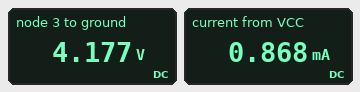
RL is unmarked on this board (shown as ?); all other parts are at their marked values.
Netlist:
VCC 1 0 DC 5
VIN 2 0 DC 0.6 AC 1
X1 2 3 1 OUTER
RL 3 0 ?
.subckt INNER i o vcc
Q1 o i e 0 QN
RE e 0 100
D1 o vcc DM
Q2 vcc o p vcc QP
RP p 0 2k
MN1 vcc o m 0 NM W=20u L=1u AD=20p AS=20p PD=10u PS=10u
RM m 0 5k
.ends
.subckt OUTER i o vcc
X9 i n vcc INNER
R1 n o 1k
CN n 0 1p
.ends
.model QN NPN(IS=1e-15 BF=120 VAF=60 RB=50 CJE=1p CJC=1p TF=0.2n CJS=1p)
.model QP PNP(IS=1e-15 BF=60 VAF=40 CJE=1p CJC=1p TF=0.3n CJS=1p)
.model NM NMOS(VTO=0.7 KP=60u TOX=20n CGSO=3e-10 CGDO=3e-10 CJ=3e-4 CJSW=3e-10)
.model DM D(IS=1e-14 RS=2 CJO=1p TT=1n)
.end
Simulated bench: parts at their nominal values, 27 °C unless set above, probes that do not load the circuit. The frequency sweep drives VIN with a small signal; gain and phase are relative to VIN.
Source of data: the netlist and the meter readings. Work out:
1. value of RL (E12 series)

27 kΩ
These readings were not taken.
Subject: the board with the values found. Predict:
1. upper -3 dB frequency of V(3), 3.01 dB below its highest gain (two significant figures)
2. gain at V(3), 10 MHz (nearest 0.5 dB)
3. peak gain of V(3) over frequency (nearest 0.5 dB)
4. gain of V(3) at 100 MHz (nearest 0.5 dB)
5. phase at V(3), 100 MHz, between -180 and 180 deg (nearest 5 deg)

6.2 GHz
-23.5 dB
-23.0 dB
-26.0 dB
95 deg
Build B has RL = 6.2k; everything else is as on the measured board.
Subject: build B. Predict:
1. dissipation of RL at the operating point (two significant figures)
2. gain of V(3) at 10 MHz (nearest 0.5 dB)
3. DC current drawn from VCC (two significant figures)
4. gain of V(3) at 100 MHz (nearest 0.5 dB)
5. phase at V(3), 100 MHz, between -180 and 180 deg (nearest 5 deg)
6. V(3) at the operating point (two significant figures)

2.2 mW
-36.0 dB
1.7 mA
-37.0 dB
110 deg
3.7 V
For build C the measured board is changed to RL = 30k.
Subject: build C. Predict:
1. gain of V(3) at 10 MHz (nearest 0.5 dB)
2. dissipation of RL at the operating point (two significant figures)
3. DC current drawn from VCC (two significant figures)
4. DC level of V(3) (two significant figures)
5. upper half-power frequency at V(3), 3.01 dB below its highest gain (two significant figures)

-23.0 dB
590 µW
840 µA
4.2 V
5.4 GHz
